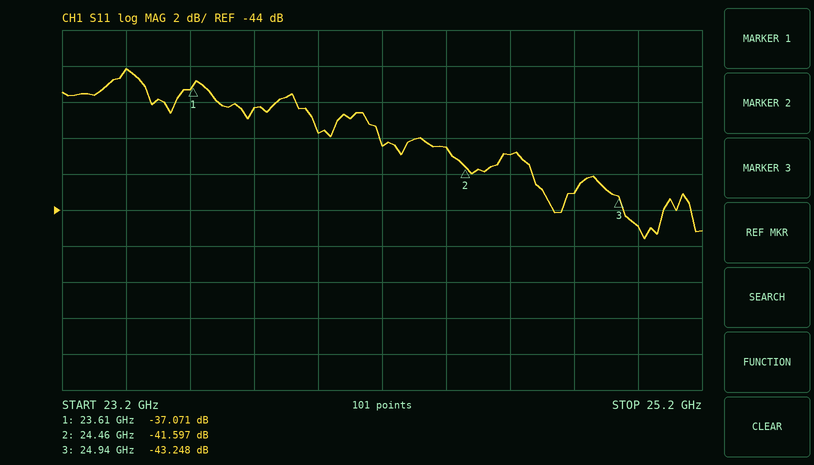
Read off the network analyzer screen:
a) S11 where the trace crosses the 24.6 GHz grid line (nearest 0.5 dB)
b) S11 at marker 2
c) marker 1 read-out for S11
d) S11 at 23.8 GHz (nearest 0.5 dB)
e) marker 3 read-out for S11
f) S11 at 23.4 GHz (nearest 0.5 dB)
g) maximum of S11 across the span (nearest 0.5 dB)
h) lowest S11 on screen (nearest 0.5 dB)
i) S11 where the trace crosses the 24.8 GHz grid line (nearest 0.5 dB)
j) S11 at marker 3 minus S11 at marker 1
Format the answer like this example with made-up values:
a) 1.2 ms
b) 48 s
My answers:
a) -41.0 dB
b) -41.597 dB
c) -37.071 dB
d) -38.5 dB
e) -43.248 dB
f) -36.0 dB
g) -36.0 dB
h) -45.5 dB
i) -43.0 dB
j) -6.177 dB
